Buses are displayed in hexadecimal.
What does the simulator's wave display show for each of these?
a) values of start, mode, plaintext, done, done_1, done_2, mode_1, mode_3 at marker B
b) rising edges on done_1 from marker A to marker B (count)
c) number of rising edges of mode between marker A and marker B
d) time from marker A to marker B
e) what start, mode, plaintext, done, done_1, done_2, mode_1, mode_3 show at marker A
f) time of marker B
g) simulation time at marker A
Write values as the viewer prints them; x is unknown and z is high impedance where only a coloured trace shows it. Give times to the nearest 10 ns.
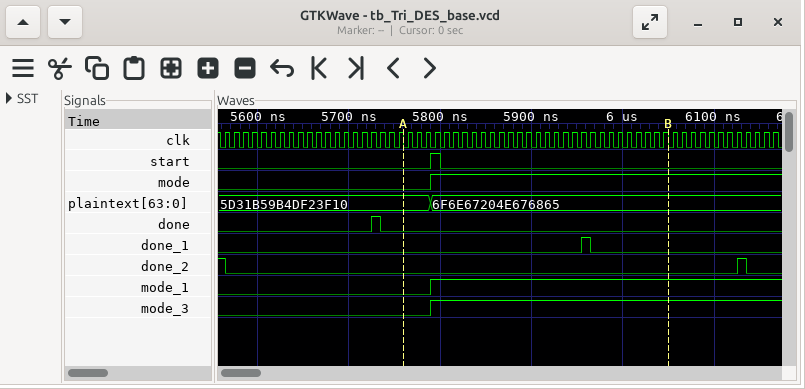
start=0, mode=1, plaintext=6F6E67204E676865, done=0, done_1=0, done_2=0, mode_1=1, mode_3=1
1
1
290 ns
start=0, mode=0, plaintext=5D31B59B4DF23F10, done=0, done_1=0, done_2=0, mode_1=0, mode_3=0
6050 ns
5760 ns
